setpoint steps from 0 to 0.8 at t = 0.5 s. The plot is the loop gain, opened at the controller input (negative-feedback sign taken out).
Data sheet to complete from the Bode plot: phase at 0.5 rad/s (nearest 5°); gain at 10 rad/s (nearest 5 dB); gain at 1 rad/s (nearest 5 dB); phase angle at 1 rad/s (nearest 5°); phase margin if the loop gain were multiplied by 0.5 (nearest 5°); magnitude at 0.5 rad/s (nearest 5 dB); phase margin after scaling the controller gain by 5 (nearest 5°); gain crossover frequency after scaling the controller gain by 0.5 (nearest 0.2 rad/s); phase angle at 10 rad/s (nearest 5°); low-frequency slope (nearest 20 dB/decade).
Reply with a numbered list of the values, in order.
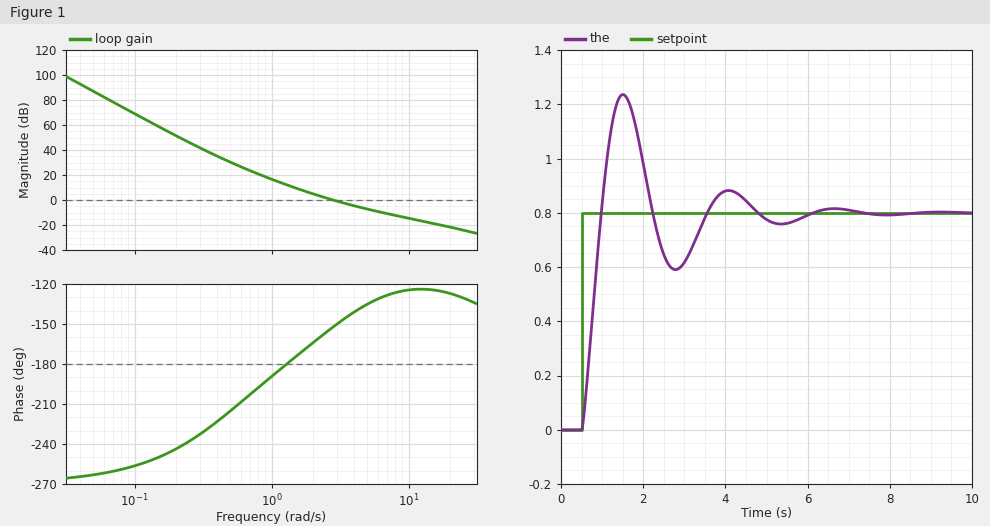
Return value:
1. -215°
2. -15 dB
3. 15 dB
4. -190°
5. 15°
6. 30 dB
7. 55°
8. 1.8 rad/s
9. -125°
10. -60 dB/decade
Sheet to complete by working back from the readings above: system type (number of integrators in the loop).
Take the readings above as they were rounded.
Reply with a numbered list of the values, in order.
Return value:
1. 3
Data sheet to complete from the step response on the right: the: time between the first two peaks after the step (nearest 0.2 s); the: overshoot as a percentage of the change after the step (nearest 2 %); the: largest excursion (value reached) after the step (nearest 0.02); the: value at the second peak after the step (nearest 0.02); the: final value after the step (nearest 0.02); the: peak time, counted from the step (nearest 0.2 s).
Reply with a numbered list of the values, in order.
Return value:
1. 2.6 s
2. 54 %
3. 1.24
4. 0.88
5. 0.80
6. 1.0 s
